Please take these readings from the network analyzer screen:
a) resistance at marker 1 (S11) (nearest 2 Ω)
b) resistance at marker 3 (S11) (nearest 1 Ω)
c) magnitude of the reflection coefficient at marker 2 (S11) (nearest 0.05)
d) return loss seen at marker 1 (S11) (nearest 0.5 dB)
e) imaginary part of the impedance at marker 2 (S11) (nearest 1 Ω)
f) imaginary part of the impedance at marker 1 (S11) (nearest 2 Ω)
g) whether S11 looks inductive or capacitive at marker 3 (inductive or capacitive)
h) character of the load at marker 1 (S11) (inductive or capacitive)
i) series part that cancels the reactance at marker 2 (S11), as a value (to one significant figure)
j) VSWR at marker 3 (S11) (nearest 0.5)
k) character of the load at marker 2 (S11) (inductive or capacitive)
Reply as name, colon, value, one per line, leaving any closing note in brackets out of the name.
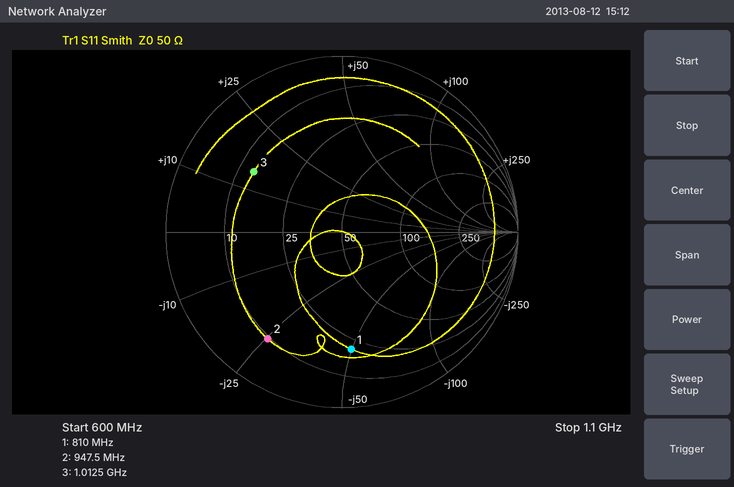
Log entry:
resistance at marker 1 (S11): 20 Ω
resistance at marker 3 (S11): 13 Ω
magnitude of the reflection coefficient at marker 2 (S11): 0.75
return loss seen at marker 1 (S11): 3.5 dB
imaginary part of the impedance at marker 2 (S11): -25 Ω
imaginary part of the impedance at marker 1 (S11): -50 Ω
whether S11 looks inductive or capacitive at marker 3: inductive
character of the load at marker 1 (S11): capacitive
series part that cancels the reactance at marker 2 (S11), as a value: 4 nH
VSWR at marker 3 (S11): 4.0
character of the load at marker 2 (S11): capacitive
